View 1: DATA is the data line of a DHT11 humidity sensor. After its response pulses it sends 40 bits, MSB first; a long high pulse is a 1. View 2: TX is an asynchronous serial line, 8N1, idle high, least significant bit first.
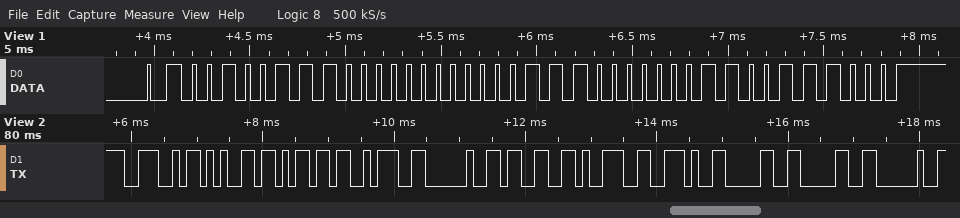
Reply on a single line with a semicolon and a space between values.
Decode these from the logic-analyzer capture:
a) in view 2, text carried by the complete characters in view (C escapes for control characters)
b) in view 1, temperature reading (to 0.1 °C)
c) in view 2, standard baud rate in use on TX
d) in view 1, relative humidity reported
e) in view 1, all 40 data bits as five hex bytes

"Nem: 39.00 "; 14.3 °C; 9600 baud; 39 %; 27 00 0E 03 38
